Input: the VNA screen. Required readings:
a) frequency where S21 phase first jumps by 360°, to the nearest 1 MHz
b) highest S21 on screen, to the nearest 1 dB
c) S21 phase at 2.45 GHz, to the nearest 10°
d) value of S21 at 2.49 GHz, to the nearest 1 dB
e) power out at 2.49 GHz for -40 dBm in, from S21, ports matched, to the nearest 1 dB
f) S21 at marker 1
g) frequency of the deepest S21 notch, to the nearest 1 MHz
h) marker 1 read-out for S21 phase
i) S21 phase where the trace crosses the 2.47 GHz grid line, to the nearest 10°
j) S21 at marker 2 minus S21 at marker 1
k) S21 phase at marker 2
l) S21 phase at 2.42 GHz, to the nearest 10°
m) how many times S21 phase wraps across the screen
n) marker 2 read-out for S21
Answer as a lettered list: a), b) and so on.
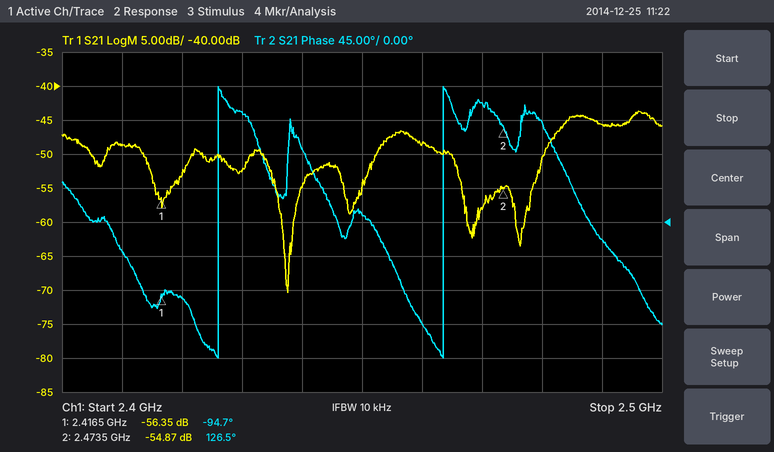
a) 2.426 GHz
b) -44 dB
c) 10°
d) -46 dB
e) -86 dBm
f) -56.35 dB
g) 2.438 GHz
h) -94.7°
i) 160°
j) 1.48 dB
k) 126.5°
l) -100°
m) 2
n) -54.87 dB
